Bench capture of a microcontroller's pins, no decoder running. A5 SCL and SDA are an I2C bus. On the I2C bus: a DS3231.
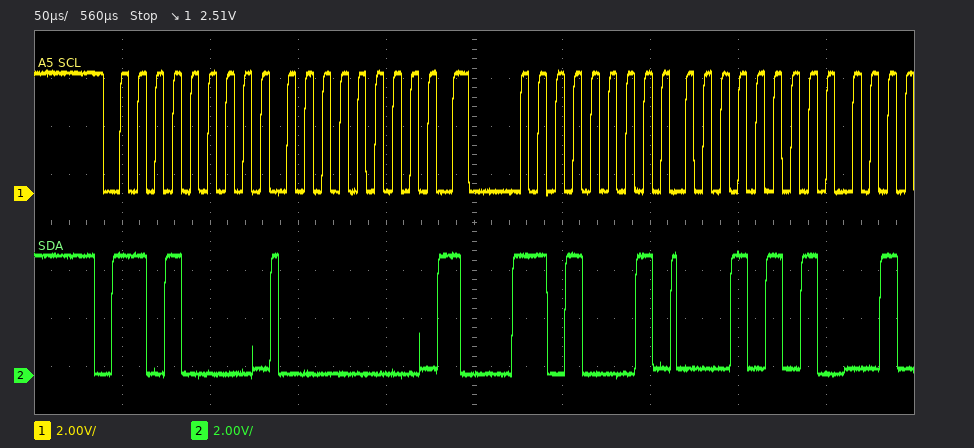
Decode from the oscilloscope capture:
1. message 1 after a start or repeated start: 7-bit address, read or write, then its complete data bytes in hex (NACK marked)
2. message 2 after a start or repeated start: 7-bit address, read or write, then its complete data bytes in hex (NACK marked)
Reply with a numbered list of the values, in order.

1. 0x68 write: 00
2. 0x68 read: 15
